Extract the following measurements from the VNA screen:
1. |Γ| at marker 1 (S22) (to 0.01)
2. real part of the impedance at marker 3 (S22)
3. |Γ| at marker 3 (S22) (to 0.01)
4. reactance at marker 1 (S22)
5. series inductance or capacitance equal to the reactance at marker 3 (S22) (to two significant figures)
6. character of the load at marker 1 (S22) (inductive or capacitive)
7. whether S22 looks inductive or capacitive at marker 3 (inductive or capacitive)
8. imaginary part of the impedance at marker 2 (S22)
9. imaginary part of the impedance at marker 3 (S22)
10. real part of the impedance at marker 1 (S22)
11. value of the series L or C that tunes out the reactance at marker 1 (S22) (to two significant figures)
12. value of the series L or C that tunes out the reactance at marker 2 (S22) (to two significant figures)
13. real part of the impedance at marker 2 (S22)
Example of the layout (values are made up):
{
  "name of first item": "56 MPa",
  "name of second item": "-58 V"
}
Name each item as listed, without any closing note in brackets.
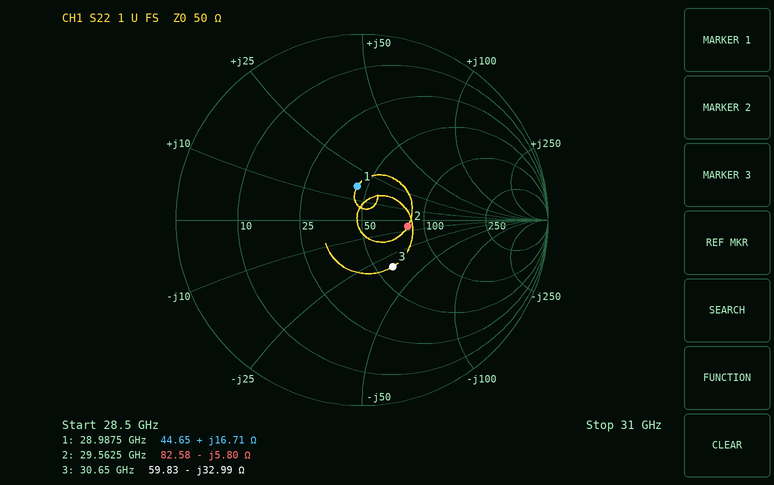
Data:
{
  "|Γ| at marker 1 (S22)": "0.18",
  "real part of the impedance at marker 3": "59.83 Ω",
  "|Γ| at marker 3 (S22)": "0.30",
  "reactance at marker 1": "+16.71 Ω",
  "series inductance or capacitance equal to the reactance at marker 3 (S22)": "160 fF",
  "character of the load at marker 1 (S22)": "inductive",
  "whether S22 looks inductive or capacitive at marker 3": "capacitive",
  "imaginary part of the impedance at marker 2": "-5.80 Ω",
  "imaginary part of the impedance at marker 3": "-32.99 Ω",
  "real part of the impedance at marker 1": "44.65 Ω",
  "value of the series L or C that tunes out the reactance at marker 1 (S22)": "330 fF",
  "value of the series L or C that tunes out the reactance at marker 2 (S22)": "31 pH",
  "real part of the impedance at marker 2": "82.58 Ω"
}
